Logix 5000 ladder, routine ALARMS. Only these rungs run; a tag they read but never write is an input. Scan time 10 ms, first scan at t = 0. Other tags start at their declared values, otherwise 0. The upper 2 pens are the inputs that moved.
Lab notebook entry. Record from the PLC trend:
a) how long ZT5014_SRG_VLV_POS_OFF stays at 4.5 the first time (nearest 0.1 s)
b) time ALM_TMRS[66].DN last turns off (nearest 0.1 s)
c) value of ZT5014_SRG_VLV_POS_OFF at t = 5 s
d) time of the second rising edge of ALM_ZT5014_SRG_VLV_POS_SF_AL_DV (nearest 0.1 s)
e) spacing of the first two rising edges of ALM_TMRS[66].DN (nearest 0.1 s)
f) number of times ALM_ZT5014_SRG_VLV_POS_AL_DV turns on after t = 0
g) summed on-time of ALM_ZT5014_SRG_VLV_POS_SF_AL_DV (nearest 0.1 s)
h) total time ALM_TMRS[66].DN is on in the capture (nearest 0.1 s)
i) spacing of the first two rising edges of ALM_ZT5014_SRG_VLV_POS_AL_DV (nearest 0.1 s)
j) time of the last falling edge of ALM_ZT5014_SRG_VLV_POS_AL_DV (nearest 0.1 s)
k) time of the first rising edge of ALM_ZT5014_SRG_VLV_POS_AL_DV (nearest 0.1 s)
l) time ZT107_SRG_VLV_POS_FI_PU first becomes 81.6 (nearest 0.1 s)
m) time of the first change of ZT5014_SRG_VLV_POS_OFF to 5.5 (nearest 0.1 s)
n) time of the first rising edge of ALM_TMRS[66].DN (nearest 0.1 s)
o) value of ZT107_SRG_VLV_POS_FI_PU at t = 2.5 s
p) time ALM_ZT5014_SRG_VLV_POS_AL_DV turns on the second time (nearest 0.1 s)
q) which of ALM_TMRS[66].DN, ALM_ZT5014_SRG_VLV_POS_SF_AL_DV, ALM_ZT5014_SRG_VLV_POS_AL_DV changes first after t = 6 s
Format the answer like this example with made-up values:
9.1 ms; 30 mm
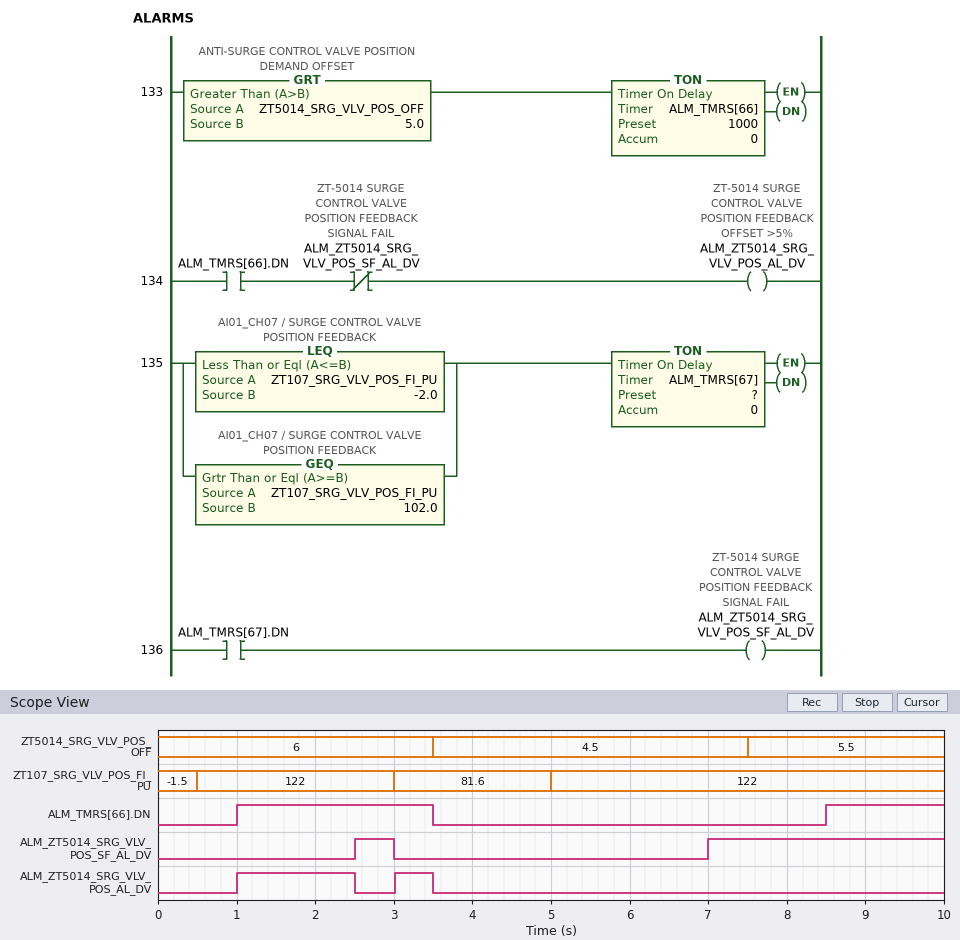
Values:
4.0 s; 3.5 s; 4.5; 7.0 s; 7.5 s; 2; 3.5 s; 4.0 s; 2.0 s; 3.5 s; 1.0 s; 3.0 s; 7.5 s; 1.0 s; 122; 3.0 s; ALM_ZT5014_SRG_VLV_POS_SF_AL_DV
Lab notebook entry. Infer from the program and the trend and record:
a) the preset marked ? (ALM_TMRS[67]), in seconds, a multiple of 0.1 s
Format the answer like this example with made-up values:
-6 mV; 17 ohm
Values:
2.0 s
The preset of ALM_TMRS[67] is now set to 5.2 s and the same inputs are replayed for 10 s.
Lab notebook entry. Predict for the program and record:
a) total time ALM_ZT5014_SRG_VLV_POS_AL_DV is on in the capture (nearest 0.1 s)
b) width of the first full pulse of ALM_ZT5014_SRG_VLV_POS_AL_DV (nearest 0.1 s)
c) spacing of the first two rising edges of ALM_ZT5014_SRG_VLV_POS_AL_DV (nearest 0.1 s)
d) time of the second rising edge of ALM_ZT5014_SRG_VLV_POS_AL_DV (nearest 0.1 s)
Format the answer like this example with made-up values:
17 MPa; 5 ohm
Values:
4.0 s; 2.5 s; 7.5 s; 8.5 s
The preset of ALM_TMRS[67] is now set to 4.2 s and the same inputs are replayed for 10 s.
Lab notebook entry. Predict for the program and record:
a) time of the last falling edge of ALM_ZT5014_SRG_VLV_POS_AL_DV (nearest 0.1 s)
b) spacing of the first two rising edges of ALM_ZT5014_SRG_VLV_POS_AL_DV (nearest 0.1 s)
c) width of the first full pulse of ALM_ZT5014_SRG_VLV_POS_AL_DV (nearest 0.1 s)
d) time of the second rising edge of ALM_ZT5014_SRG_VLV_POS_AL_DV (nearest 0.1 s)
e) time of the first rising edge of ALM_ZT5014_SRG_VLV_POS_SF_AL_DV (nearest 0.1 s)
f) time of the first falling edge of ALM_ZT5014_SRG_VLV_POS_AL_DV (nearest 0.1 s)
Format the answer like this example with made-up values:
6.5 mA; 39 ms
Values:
9.2 s; 7.5 s; 2.5 s; 8.5 s; 9.2 s; 3.5 s
